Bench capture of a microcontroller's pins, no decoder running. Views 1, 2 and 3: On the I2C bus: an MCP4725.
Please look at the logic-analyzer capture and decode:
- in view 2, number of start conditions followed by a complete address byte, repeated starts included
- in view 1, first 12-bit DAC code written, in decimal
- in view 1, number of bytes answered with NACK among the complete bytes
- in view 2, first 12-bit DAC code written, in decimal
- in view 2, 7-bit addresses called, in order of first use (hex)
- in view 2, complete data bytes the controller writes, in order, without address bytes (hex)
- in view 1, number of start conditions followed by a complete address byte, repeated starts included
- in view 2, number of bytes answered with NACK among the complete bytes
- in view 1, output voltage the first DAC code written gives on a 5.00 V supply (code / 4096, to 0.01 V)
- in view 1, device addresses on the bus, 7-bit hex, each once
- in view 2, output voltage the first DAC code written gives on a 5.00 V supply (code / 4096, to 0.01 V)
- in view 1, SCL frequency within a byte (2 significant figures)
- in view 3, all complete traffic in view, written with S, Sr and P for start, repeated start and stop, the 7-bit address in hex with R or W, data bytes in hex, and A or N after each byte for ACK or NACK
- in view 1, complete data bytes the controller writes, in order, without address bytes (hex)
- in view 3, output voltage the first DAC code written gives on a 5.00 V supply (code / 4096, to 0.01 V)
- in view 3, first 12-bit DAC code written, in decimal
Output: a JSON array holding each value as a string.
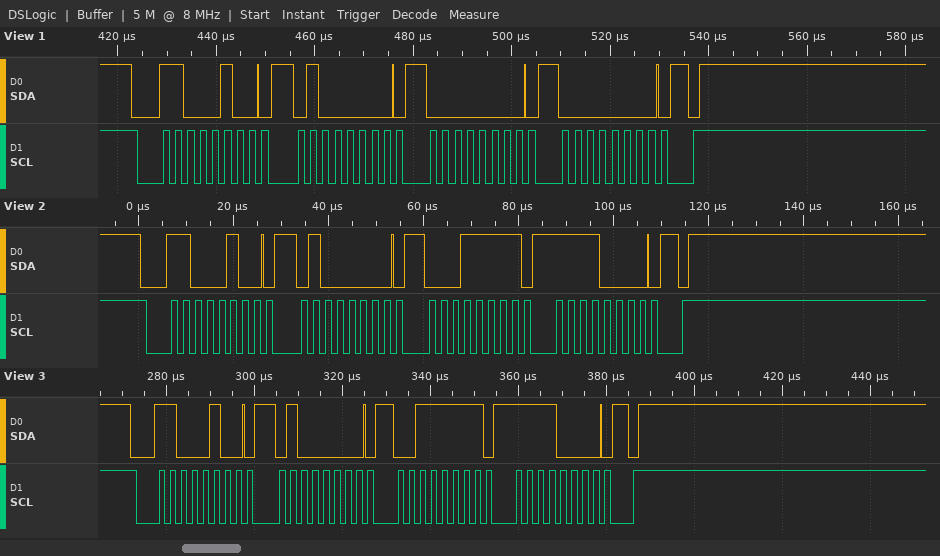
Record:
["1", "0", "0", "511", "0x62", "40 1F F0", "1", "0", "0.00 V", "0x62", "0.62 V", "400 kHz", "S 62W A 40 A 3F A F0 A P", "40 00 00", "1.25 V", "1023"]
